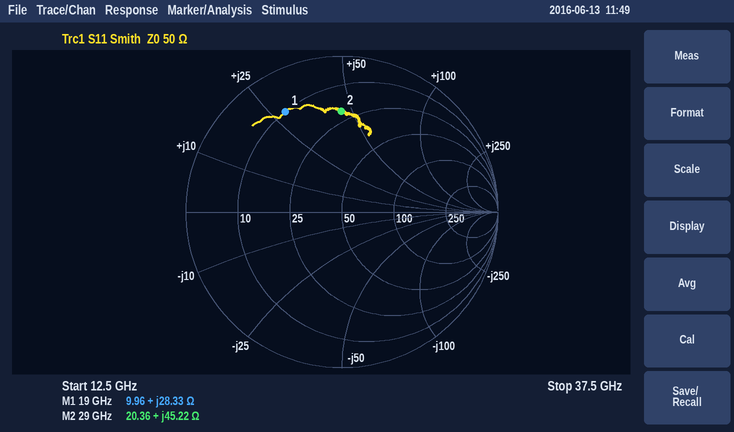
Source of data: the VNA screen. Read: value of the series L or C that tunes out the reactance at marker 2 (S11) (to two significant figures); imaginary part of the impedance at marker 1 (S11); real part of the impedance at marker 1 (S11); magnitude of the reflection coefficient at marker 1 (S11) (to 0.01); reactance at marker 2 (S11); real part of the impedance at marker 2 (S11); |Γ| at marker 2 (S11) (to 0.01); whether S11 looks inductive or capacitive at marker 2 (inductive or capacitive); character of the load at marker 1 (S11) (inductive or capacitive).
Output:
120 fF
+28.33 Ω
9.96 Ω
0.74
+45.22 Ω
20.36 Ω
0.65
inductive
inductive
